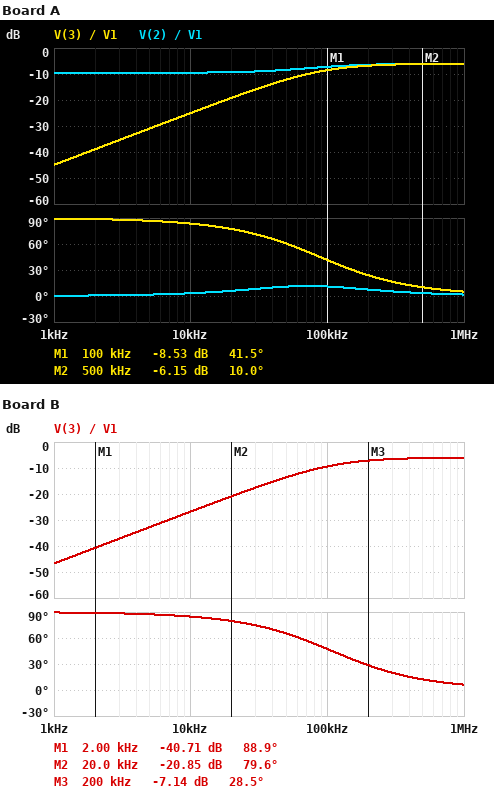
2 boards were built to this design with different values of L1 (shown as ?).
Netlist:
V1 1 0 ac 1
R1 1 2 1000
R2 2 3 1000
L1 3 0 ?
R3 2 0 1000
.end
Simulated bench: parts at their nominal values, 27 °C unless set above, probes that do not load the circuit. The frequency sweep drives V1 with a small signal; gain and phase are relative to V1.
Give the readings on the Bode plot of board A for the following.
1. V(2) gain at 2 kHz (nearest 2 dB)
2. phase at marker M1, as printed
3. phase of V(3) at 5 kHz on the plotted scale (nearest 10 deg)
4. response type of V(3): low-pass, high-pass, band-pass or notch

-10 dB
41.5 deg
90 deg
high-pass
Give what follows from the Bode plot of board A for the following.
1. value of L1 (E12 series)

2.7 mH
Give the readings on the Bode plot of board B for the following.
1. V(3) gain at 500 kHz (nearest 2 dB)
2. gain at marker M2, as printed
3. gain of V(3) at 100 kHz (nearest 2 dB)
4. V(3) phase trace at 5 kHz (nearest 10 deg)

-6 dB
-20.85 dB
-10 dB
90 deg
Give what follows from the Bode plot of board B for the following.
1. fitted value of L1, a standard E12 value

2.2 mH
